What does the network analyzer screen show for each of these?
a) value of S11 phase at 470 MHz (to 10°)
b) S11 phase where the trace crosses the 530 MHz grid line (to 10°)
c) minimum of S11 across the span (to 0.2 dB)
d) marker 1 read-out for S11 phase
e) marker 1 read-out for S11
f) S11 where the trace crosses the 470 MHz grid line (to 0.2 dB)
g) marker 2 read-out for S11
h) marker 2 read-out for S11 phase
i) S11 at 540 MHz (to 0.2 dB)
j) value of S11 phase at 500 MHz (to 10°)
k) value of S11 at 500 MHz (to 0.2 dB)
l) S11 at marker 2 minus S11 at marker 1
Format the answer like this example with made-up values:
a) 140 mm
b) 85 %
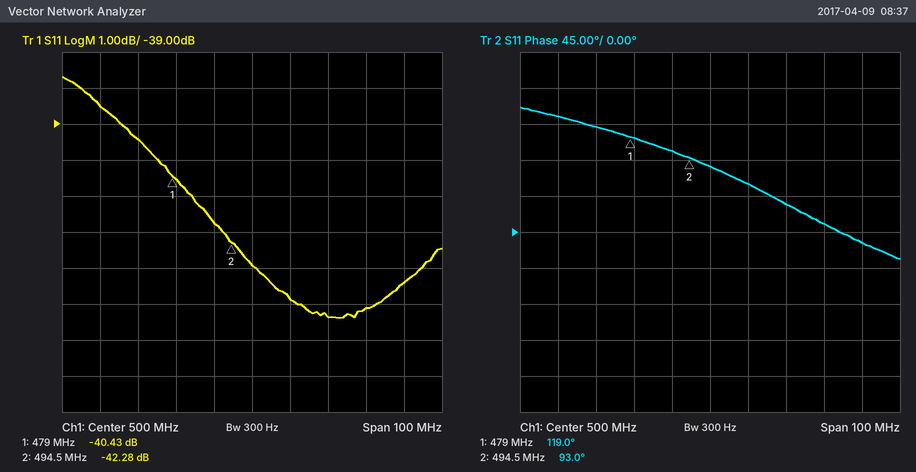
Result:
a) 130°
b) 10°
c) -44.4 dB
d) 119.0°
e) -40.43 dB
f) -39.4 dB
g) -42.28 dB
h) 93.0°
i) -43.4 dB
j) 80°
k) -43.0 dB
l) -1.85 dB
